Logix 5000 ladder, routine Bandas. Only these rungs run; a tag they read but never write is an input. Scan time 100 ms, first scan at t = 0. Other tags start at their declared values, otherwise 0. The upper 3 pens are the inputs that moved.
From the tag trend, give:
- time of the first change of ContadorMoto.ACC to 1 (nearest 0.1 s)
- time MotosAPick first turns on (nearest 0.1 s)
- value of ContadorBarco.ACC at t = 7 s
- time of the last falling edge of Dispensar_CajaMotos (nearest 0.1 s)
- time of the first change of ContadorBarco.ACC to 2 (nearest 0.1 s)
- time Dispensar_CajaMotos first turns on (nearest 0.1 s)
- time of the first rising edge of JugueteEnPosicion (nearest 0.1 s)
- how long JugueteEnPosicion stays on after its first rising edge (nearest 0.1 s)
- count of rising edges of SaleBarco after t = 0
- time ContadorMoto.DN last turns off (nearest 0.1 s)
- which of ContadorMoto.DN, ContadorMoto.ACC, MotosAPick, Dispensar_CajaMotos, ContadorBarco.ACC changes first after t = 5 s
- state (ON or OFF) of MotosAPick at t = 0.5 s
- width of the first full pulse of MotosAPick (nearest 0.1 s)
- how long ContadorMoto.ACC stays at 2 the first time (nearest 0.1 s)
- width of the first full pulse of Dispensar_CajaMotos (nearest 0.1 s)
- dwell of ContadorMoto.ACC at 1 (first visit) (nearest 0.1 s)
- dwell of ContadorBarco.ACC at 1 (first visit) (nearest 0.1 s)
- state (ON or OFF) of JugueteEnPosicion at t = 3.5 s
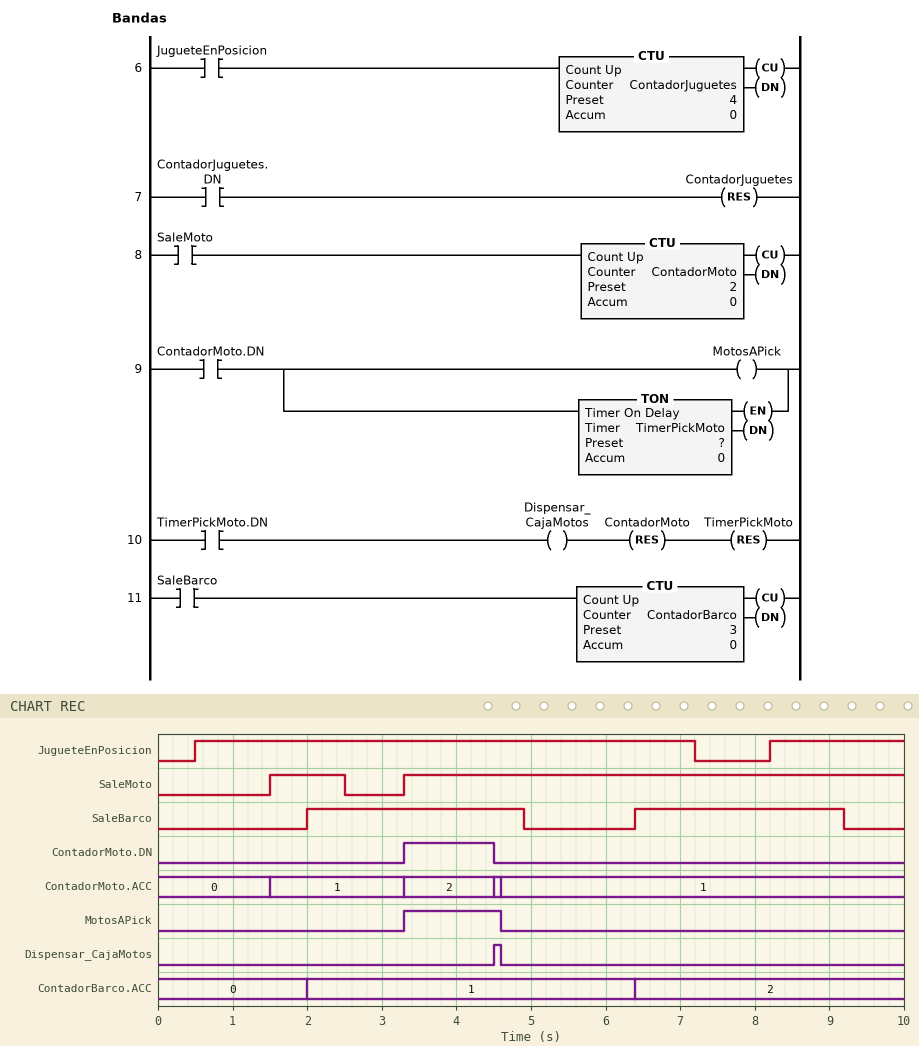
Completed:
1.5 s
3.3 s
2
4.6 s
6.4 s
4.5 s
0.5 s
6.7 s
2
4.5 s
ContadorBarco.ACC
OFF
1.3 s
1.2 s
0.1 s
1.8 s
4.4 s
ON
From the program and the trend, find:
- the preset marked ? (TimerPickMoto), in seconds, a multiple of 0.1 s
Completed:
1.2 s
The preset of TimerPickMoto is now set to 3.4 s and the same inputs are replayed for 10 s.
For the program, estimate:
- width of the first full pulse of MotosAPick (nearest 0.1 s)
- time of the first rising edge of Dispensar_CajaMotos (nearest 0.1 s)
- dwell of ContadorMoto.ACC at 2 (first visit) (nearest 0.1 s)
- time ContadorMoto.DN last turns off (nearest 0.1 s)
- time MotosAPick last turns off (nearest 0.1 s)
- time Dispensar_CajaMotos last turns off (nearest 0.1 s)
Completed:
3.5 s
6.7 s
3.4 s
6.7 s
6.8 s
6.8 s
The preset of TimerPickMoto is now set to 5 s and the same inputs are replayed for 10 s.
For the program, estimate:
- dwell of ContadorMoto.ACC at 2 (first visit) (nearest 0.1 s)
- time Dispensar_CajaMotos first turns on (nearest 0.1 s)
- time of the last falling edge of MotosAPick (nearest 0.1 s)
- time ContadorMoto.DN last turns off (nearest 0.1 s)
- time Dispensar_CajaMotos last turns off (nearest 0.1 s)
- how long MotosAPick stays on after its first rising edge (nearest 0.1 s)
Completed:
5.0 s
8.3 s
8.4 s
8.3 s
8.4 s
5.1 s
